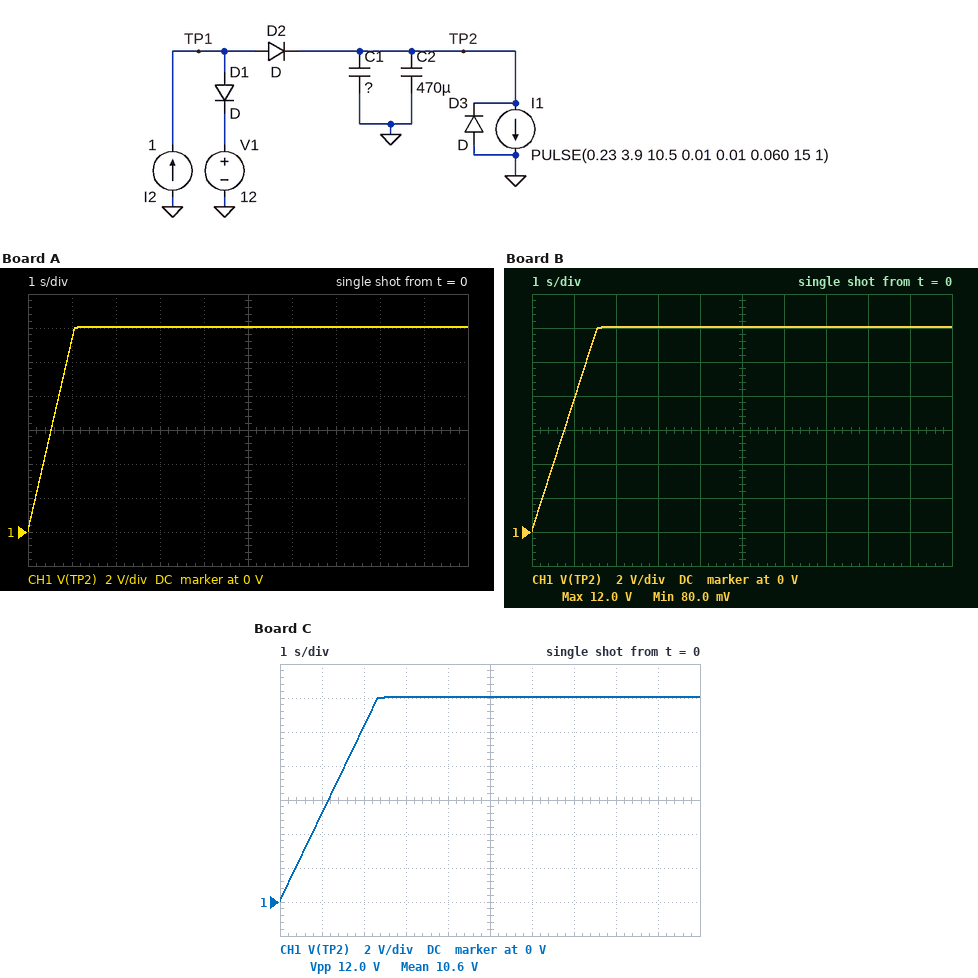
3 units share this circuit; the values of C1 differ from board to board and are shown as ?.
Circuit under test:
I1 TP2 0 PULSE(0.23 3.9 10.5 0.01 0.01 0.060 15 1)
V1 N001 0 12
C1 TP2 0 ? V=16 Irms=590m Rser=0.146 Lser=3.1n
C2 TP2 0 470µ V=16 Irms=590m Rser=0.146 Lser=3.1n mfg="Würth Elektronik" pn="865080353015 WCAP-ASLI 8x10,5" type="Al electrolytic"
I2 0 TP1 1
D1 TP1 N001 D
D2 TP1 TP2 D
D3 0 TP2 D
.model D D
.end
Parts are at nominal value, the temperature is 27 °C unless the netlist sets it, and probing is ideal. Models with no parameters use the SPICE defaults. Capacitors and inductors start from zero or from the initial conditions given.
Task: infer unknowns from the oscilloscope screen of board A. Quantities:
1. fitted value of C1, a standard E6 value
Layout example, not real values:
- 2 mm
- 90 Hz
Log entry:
- 68 mF
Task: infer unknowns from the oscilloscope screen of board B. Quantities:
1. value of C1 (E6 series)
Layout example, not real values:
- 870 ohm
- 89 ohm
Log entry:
- 100 mF
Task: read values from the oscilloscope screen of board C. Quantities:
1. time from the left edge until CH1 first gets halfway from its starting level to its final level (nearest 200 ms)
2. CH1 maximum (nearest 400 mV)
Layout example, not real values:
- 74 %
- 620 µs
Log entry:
- 1.2 s
- 12.0 V
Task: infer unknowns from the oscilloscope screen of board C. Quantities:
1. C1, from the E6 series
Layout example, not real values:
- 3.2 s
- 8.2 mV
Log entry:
- 150 mF
